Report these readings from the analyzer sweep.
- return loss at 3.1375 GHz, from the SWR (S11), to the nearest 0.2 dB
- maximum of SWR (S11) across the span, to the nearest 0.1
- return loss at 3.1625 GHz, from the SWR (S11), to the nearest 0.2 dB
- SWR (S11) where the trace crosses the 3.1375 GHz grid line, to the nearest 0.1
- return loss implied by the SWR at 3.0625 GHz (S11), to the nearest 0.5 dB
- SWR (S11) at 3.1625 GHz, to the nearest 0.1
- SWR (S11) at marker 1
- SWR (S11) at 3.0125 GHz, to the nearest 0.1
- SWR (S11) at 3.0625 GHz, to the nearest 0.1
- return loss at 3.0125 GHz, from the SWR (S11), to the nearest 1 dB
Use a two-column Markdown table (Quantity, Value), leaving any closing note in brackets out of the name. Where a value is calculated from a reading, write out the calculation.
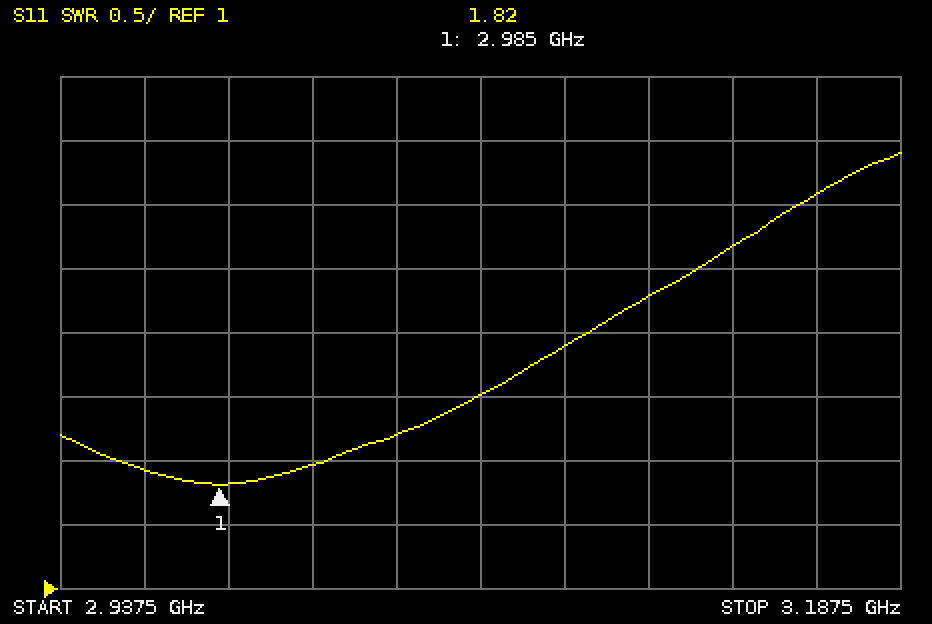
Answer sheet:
| Quantity | Value |
|---|---|
| return loss at 3.1375 GHz, from the SWR (S11), to the nearest 0.2 dB | −20 log10((3.7 − 1)/(3.7 + 1)) ≈ 4.8 dB |
| maximum of SWR (S11) across the span, to the nearest 0.1 | 4.4 |
| return loss at 3.1625 GHz, from the SWR (S11), to the nearest 0.2 dB | −20 log10((4.1 − 1)/(4.1 + 1)) ≈ 4.32 dB, so 4.4 dB to the nearest 0.2 dB |
| SWR (S11) where the trace crosses the 3.1375 GHz grid line, to the nearest 0.1 | 3.7 |
| return loss implied by the SWR at 3.0625 GHz (S11), to the nearest 0.5 dB | −20 log10((2.5 − 1)/(2.5 + 1)) ≈ 7.36 dB, so 7.5 dB to the nearest 0.5 dB |
| SWR (S11) at 3.1625 GHz, to the nearest 0.1 | 4.1 |
| SWR (S11) at marker 1 | 1.82 |
| SWR (S11) at 3.0125 GHz, to the nearest 0.1 | 2.0 |
| SWR (S11) at 3.0625 GHz, to the nearest 0.1 | 2.5 |
| return loss at 3.0125 GHz, from the SWR (S11), to the nearest 1 dB | −20 log10((2 − 1)/(2 + 1)) ≈ 10 dB |
